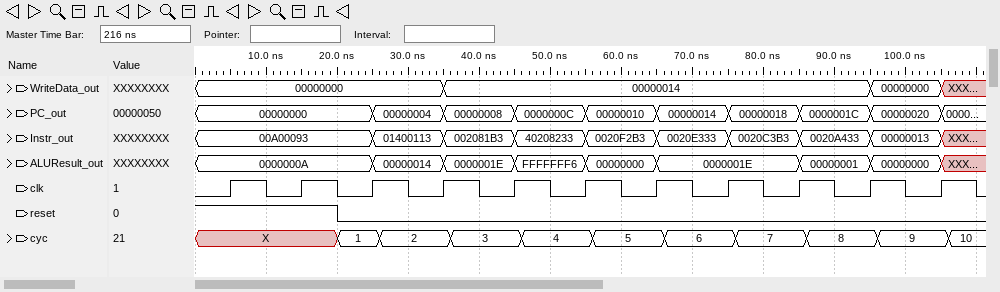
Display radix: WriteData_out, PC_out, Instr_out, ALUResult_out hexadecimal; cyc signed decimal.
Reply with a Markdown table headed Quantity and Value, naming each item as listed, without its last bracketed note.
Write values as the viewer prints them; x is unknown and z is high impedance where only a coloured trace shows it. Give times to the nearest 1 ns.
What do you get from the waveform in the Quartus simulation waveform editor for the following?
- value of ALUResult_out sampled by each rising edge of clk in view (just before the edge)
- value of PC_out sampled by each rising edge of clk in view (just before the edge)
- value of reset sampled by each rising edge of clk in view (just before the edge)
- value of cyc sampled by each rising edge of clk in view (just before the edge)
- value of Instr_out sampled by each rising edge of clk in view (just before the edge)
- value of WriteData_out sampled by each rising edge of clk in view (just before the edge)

| Quantity | Value |
|---|---|
| value of ALUResult_out sampled by each rising edge of clk in view | 0000000A, 0000000A, 0000000A, 00000014, 0000001E, FFFFFFF6, 00000000, 0000001E, 0000001E, 00000001, 00000000 |
| value of PC_out sampled by each rising edge of clk in view | 00000000, 00000000, 00000000, 00000004, 00000008, 0000000C, 00000010, 00000014, 00000018, 0000001C, 00000020 |
| value of reset sampled by each rising edge of clk in view | 1 1 0 0 0 0 0 0 0 0 0 |
| value of cyc sampled by each rising edge of clk in view | X, X, 1, 2, 3, 4, 5, 6, 7, 8, 9 |
| value of Instr_out sampled by each rising edge of clk in view | 00A00093, 00A00093, 00A00093, 01400113, 002081B3, 40208233, 0020F2B3, 0020E333, 0020C3B3, 0020A433, 00000013 |
| value of WriteData_out sampled by each rising edge of clk in view | 00000000, 00000000, 00000000, 00000000, 00000014, 00000014, 00000014, 00000014, 00000014, 00000014, 00000000 |
